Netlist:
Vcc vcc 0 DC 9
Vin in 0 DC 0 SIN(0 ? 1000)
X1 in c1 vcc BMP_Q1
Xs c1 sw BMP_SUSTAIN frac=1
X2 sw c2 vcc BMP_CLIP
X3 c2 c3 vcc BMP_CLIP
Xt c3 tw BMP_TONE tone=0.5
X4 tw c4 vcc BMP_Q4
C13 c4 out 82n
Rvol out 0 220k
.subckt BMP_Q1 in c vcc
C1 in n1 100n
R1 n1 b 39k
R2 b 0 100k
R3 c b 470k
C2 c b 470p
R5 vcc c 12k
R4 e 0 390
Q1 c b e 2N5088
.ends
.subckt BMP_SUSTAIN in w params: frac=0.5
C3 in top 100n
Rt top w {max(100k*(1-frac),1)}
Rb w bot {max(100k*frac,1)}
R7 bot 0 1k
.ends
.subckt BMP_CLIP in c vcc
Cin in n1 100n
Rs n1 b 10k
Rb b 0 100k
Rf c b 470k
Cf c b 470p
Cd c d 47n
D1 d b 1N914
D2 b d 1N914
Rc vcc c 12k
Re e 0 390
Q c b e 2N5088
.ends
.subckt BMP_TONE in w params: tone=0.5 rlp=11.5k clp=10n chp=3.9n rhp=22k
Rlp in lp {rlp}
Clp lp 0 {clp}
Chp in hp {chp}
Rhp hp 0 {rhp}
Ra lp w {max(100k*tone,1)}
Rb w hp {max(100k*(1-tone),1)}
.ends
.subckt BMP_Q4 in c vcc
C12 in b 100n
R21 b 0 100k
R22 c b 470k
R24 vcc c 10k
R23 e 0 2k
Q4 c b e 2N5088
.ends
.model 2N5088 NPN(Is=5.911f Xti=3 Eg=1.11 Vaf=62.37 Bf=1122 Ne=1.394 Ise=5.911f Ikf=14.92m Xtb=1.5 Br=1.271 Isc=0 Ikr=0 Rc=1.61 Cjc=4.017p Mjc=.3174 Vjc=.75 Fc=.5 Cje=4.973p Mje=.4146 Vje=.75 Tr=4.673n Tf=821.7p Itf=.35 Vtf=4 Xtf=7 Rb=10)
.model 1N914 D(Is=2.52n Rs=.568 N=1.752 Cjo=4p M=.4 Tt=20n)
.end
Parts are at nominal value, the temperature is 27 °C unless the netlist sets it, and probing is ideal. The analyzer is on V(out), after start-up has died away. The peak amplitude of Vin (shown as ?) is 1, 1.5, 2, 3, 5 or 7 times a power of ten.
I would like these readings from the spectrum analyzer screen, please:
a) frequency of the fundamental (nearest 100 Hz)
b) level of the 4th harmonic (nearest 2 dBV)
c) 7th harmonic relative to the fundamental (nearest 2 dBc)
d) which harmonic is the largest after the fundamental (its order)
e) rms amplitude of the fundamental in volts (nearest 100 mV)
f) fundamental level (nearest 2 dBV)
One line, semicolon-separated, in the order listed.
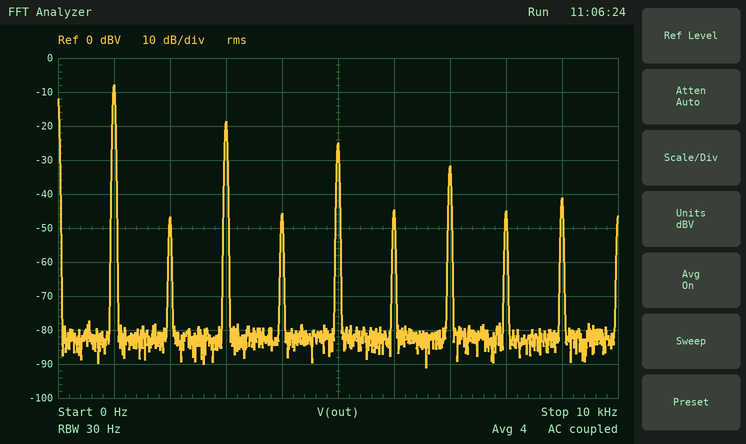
1.0 kHz; -46 dBV; -24 dBc; 3; 400 mV; -8 dBV
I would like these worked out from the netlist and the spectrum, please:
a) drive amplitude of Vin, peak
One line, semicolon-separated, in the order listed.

500 mV
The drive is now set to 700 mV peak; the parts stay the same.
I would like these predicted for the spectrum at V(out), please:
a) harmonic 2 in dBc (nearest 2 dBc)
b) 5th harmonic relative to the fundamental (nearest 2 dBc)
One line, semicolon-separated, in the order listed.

-42 dBc; -20 dBc
